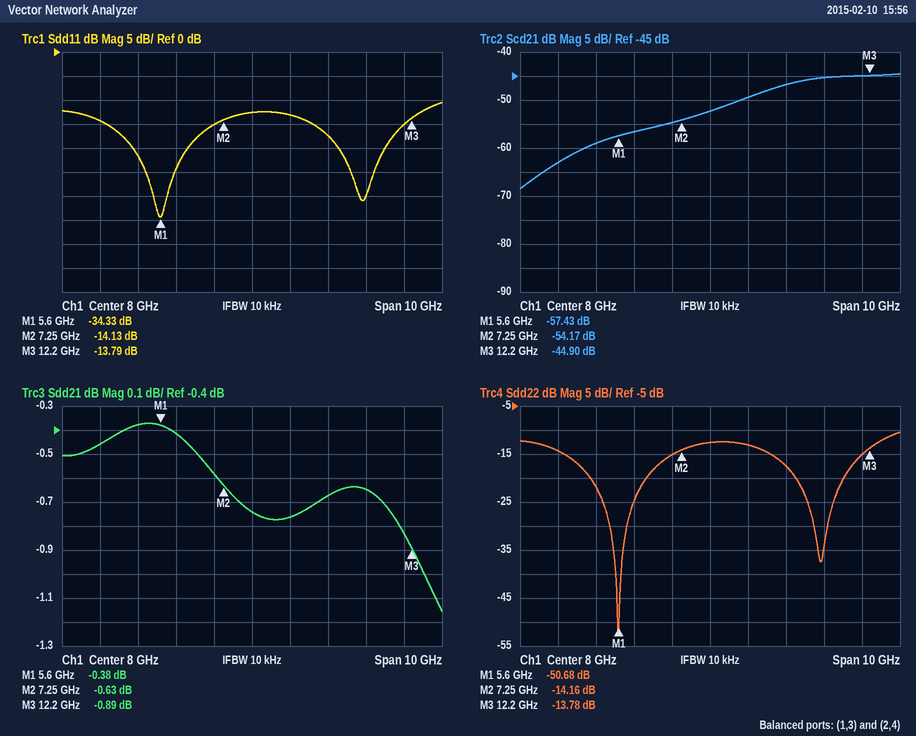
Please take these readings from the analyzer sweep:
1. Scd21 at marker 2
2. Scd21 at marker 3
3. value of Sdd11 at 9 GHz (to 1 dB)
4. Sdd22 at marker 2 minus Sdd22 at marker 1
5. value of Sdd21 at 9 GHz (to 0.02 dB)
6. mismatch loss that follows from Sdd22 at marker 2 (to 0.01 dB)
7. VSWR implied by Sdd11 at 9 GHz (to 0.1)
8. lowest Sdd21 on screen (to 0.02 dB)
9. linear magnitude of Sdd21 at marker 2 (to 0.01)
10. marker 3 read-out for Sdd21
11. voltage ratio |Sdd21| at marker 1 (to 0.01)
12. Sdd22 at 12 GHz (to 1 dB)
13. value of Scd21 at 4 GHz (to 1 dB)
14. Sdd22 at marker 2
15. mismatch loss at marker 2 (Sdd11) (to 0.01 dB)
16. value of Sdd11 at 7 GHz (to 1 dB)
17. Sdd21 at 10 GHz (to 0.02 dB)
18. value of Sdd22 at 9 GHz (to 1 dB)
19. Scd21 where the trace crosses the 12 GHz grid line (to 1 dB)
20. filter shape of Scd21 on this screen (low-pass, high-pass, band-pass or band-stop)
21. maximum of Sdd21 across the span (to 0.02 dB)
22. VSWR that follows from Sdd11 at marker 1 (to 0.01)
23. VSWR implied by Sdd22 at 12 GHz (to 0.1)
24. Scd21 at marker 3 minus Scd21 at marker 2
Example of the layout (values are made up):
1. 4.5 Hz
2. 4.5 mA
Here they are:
1. -54.17 dB
2. -44.90 dB
3. -13 dB
4. 36.52 dB
5. -0.76 dB
6. 0.17 dB
7. 1.6
8. -1.16 dB
9. 0.93
10. -0.89 dB
11. 0.96
12. -15 dB
13. -63 dB
14. -14.16 dB
15. 0.17 dB
16. -15 dB
17. -0.68 dB
18. -13 dB
19. -45 dB
20. high-pass
21. -0.38 dB
22. 1.04
23. 1.4
24. 9.27 dB
